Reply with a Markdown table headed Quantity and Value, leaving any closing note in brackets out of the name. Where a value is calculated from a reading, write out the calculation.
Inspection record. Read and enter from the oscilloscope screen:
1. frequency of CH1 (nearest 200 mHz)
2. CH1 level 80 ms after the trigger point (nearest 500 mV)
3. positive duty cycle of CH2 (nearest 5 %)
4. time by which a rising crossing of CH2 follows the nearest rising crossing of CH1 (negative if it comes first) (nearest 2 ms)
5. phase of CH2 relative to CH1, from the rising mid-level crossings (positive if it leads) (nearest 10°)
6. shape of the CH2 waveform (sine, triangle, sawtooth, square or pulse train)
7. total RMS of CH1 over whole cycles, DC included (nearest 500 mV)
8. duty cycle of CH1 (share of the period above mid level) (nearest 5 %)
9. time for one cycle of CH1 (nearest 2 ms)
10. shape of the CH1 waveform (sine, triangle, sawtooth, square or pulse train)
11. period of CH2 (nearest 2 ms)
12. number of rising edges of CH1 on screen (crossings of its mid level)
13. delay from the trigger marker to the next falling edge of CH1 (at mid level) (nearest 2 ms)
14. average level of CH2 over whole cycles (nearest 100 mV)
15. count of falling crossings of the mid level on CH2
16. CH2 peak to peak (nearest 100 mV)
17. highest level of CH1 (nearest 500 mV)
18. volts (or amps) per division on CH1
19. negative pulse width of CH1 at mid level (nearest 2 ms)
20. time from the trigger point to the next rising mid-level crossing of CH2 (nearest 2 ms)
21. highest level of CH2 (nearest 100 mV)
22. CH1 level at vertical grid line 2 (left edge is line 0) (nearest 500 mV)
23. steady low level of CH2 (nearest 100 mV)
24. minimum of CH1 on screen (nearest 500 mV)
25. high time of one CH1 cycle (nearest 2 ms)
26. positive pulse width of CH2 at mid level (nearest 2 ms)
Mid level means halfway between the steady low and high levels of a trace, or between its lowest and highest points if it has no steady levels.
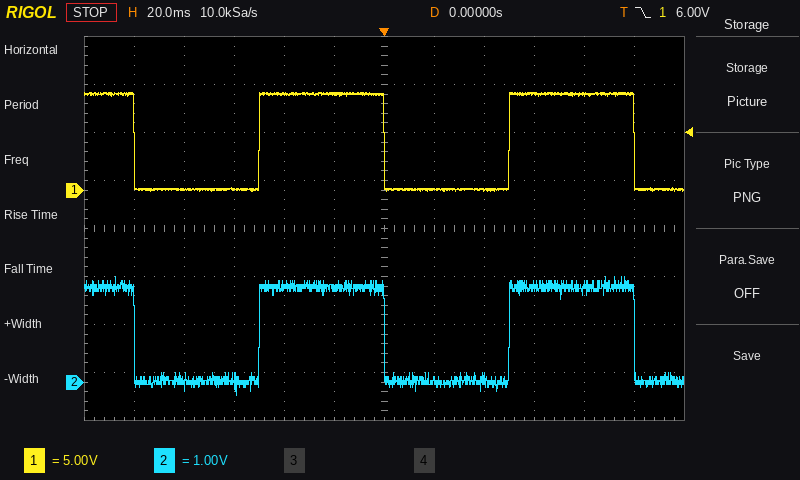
| Quantity | Value |
|---|---|
| frequency of CH1 | 1 / 100 ms ≈ 10.0 Hz |
| CH1 level 80 ms after the trigger point | 10.0 V |
| positive duty cycle of CH2 | 50 ms / 100 ms ≈ 50 % |
| time by which a rising crossing of CH2 follows the nearest rising crossing of CH1 (negative if it comes first) | 0 ms |
| phase of CH2 relative to CH1, from the rising mid-level crossings (positive if it leads) | −360° × (0 ms) / 100 ms ≈ 0° |
| shape of the CH2 waveform | square |
| total RMS of CH1 over whole cycles, DC included | √(0.5 × (10.0 V)² + 0.5 × (0.0 V)²) ≈ 7.07 V, so 7.0 V to the nearest 500 mV |
| duty cycle of CH1 (share of the period above mid level) | 50 ms / 100 ms ≈ 50 % |
| time for one cycle of CH1 | 100 ms |
| shape of the CH1 waveform | square |
| period of CH2 | 100 ms |
| number of rising edges of CH1 on screen | 2 |
| delay from the trigger marker to the next falling edge of CH1 (at mid level) | 100 ms |
| average level of CH2 over whole cycles | 0.0 V + 0.5 × (2.0 V − (0.0 V)) ≈ 1.0 V |
| count of falling crossings of the mid level on CH2 | 3 |
| CH2 peak to peak | 2.2 V − (-300 mV) = 2.5 V |
| highest level of CH1 | 10.0 V |
| volts (or amps) per division on CH1 | 5 V |
| negative pulse width of CH1 at mid level | 50 ms |
| time from the trigger point to the next rising mid-level crossing of CH2 | 50 ms |
| highest level of CH2 | 2.2 V |
| CH1 level at vertical grid line 2 (left edge is line 0) | 0.0 V |
| steady low level of CH2 | 0.0 V |
| minimum of CH1 on screen | 0.0 V |
| high time of one CH1 cycle | 50 ms |
| positive pulse width of CH2 at mid level | 50 ms |
